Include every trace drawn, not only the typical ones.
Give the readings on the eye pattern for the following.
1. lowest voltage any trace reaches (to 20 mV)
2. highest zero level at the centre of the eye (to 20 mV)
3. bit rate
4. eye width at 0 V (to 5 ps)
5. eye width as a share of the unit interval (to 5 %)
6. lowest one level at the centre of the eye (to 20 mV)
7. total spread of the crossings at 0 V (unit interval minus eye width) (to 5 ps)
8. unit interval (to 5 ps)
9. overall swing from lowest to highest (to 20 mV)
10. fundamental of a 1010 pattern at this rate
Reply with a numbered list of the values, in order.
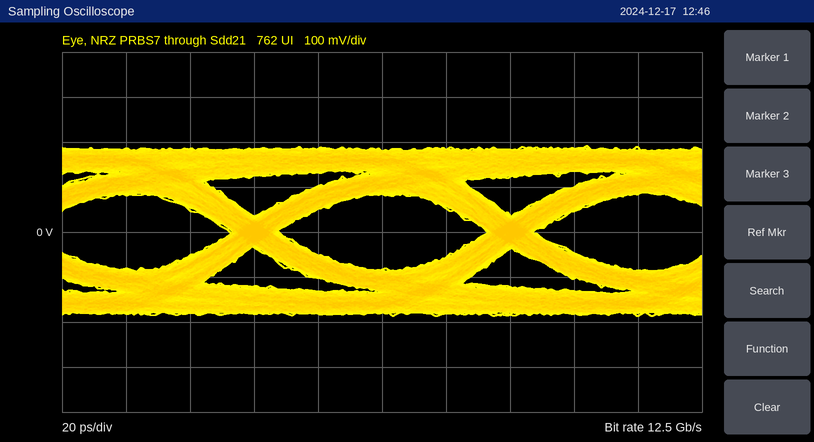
1. -180 mV
2. -80 mV
3. 12.5 Gb/s
4. 65 ps
5. 80 %
6. 80 mV
7. 15 ps
8. 80 ps
9. 380 mV
10. 6.25 GHz
